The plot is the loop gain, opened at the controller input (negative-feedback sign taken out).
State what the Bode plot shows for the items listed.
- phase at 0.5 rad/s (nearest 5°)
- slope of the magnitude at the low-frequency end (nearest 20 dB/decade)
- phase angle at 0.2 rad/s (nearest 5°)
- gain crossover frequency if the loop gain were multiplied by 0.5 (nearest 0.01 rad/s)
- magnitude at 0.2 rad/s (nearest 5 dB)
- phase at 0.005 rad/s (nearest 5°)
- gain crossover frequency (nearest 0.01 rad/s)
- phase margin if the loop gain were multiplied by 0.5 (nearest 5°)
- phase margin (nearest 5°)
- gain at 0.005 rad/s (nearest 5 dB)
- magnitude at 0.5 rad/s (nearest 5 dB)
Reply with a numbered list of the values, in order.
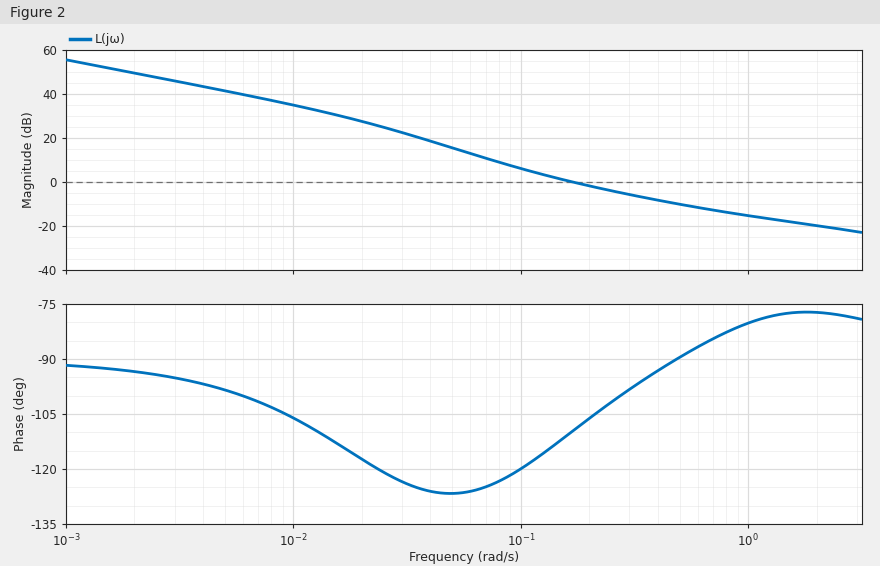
1. -90°
2. -20 dB/decade
3. -105°
4. 0.10 rad/s
5. 0 dB
6. -100°
7. 0.17 rad/s
8. 60°
9. 70°
10. 40 dB
11. -10 dB
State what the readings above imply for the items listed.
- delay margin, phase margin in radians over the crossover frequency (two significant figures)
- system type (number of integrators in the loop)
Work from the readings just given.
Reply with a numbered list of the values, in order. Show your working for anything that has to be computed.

1. 70 × π / 180 / 0.17 = 7.2 s
2. 1
